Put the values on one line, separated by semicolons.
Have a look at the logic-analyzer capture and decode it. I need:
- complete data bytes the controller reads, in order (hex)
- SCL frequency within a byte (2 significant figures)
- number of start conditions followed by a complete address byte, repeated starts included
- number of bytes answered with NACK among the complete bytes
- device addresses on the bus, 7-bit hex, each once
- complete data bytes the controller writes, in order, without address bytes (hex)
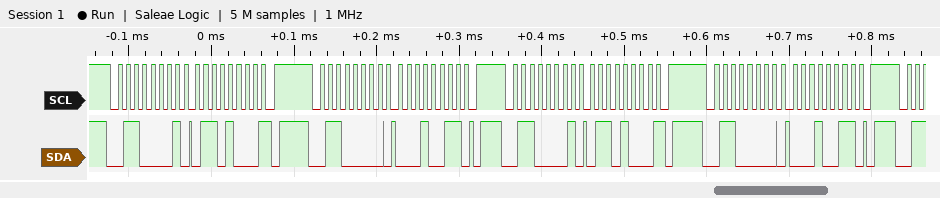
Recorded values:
68 68; 100 kHz; 4; 2; 0x30; 13 13
